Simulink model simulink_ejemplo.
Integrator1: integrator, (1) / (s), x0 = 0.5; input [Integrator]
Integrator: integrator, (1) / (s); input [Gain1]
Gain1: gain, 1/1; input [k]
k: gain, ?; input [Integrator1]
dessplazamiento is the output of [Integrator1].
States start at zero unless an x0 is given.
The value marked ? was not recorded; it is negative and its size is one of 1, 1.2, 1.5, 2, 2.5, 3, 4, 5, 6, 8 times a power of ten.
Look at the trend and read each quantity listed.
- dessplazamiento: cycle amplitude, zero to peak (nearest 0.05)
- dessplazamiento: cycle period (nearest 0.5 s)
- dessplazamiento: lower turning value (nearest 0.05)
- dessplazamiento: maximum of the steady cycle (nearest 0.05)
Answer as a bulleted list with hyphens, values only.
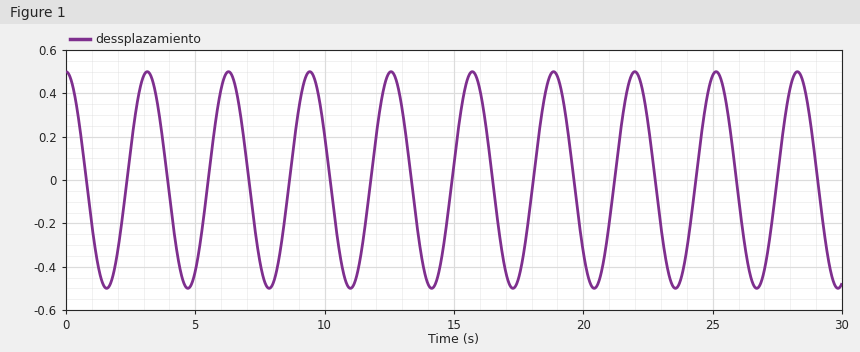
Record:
- 0.50
- 3.0 s
- -0.50
- 0.50
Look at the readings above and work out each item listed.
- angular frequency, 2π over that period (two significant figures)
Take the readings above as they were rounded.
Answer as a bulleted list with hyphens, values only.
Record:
- 2.1 rad/s
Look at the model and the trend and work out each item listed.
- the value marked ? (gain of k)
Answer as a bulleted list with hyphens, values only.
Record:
- -4
